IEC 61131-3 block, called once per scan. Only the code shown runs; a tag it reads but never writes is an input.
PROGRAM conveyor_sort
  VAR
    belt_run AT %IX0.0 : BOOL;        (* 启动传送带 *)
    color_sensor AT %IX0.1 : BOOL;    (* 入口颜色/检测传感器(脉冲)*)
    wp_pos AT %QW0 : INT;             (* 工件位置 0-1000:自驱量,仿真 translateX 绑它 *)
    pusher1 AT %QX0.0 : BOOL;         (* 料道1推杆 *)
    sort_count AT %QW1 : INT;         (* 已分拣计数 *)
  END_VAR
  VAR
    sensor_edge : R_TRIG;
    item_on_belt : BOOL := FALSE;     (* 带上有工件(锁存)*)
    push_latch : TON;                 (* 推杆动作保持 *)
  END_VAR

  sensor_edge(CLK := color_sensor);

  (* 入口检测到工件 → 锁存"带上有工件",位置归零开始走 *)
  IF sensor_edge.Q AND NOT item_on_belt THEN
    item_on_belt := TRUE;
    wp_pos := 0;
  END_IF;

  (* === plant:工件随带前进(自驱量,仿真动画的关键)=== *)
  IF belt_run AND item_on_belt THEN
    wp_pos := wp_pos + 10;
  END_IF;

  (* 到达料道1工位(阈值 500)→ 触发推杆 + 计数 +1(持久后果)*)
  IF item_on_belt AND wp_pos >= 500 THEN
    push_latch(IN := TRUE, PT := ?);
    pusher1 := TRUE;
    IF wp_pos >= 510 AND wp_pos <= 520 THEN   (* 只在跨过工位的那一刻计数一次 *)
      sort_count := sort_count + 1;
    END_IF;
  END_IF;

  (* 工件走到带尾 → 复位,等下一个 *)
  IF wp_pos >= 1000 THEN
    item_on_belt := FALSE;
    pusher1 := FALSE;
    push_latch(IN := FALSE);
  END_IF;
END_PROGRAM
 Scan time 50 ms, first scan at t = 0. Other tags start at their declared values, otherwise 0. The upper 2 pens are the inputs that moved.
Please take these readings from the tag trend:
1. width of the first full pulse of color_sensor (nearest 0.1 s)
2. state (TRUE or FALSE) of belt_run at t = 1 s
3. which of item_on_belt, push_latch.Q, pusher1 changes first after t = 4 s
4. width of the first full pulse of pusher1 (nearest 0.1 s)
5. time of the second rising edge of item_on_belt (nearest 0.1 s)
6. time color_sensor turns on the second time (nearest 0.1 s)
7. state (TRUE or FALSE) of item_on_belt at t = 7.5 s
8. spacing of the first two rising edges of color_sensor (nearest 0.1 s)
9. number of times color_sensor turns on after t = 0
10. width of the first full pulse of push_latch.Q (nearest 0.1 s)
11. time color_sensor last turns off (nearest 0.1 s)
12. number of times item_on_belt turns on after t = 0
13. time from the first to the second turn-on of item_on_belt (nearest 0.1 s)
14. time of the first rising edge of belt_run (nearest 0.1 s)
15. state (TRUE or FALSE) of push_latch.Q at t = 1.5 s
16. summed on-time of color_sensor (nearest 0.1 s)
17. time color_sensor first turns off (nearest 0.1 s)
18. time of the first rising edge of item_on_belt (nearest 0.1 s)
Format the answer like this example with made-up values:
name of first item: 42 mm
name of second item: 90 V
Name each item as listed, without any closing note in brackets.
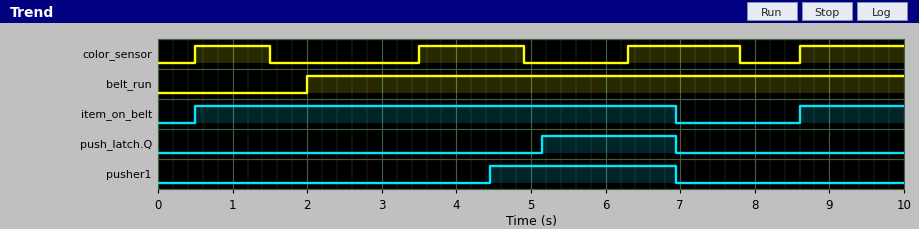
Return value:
width of the first full pulse of color_sensor: 1.0 s
state (TRUE or FALSE) of belt_run at t = 1 s: FALSE
which of item_on_belt, push_latch.Q, pusher1 changes first after t = 4 s: pusher1
width of the first full pulse of pusher1: 2.5 s
time of the second rising edge of item_on_belt: 8.6 s
time color_sensor turns on the second time: 3.5 s
state (TRUE or FALSE) of item_on_belt at t = 7.5 s: FALSE
spacing of the first two rising edges of color_sensor: 3.0 s
number of times color_sensor turns on after t = 0: 4
width of the first full pulse of push_latch.Q: 1.8 s
time color_sensor last turns off: 7.8 s
number of times item_on_belt turns on after t = 0: 2
time from the first to the second turn-on of item_on_belt: 8.1 s
time of the first rising edge of belt_run: 2.0 s
state (TRUE or FALSE) of push_latch.Q at t = 1.5 s: FALSE
summed on-time of color_sensor: 5.3 s
time color_sensor first turns off: 1.5 s
time of the first rising edge of item_on_belt: 0.5 s
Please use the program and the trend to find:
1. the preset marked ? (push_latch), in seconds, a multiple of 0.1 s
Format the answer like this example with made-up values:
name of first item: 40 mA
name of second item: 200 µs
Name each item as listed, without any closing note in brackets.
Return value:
the preset marked ? (push_latch), in seconds, a multiple of 0.1 s: 0.7 s
